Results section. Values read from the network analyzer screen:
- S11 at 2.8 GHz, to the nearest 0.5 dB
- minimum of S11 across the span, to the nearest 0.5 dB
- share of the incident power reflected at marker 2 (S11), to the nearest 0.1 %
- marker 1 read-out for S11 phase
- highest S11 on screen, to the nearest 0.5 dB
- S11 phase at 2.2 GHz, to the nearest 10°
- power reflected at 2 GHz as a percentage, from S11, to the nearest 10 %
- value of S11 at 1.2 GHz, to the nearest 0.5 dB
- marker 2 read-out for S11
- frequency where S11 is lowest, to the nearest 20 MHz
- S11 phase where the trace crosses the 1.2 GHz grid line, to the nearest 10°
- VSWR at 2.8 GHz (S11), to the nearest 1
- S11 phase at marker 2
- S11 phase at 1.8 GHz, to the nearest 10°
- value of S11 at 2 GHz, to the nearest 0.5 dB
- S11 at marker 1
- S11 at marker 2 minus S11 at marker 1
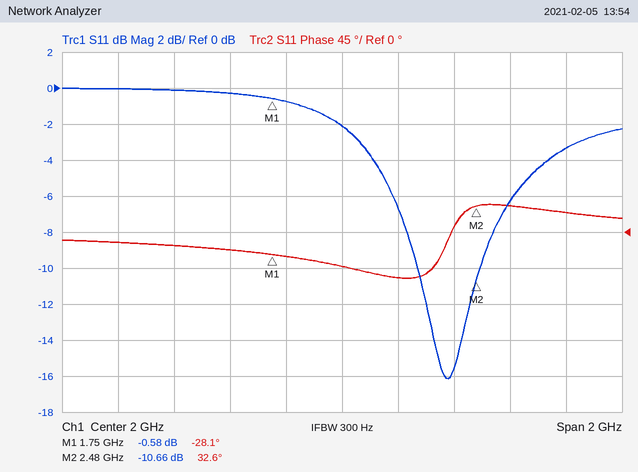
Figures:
-3.5 dB
-16.0 dB
8.6 %
-28.1°
0.0 dB
-60°
60 %
0.0 dB
-10.66 dB
2.38 GHz
-10°
5
32.6°
-30°
-2.0 dB
-0.58 dB
-10.08 dB
